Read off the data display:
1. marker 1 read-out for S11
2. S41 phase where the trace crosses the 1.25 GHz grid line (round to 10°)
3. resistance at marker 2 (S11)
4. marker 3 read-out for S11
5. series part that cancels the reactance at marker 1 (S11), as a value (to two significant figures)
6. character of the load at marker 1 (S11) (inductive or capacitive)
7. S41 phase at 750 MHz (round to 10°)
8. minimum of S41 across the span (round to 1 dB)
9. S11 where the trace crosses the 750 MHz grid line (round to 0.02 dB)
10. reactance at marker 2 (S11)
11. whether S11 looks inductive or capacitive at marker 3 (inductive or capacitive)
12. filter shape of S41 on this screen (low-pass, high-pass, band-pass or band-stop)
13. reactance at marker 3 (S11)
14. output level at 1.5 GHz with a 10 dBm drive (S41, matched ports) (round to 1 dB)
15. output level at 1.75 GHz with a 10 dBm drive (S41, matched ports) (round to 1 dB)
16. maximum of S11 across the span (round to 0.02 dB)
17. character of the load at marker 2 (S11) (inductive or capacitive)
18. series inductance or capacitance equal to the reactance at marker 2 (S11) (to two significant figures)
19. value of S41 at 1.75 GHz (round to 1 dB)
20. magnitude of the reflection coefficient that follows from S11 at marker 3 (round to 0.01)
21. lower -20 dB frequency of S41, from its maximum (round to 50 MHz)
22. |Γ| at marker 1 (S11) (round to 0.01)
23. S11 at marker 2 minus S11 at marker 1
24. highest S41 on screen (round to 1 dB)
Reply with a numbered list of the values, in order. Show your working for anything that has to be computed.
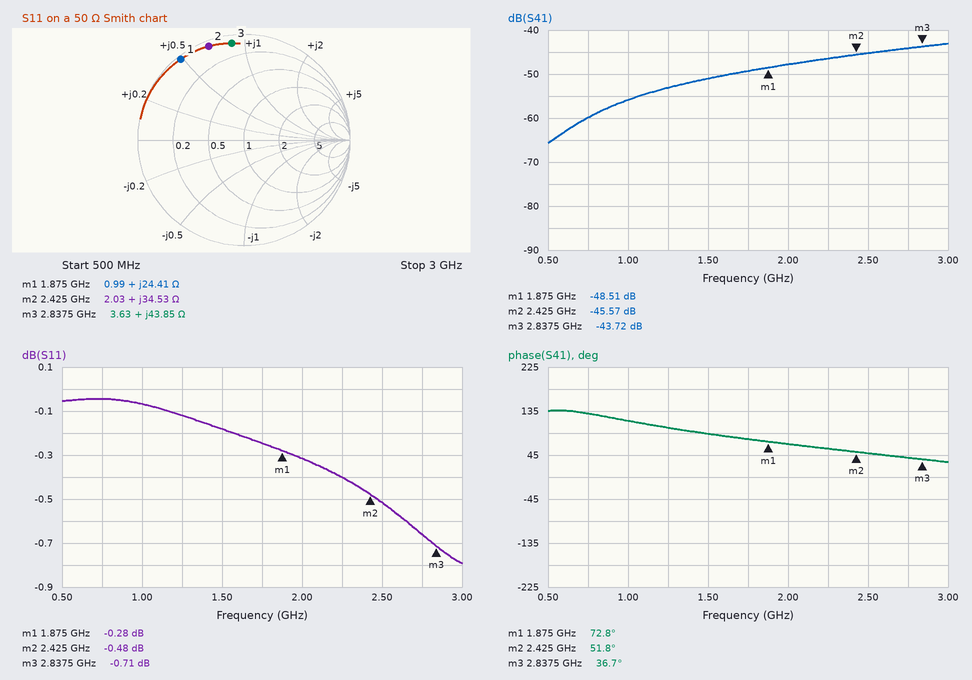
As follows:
1. -0.28 dB
2. 100°
3. 2.03 Ω
4. -0.71 dB
5. C = 1/(2π × 1.875 GHz × 24.41 Ω) ≈ 3.5 pF
6. inductive
7. 130°
8. -66 dB
9. -0.04 dB
10. +34.53 Ω
11. inductive
12. high-pass
13. +43.85 Ω
14. 10 dBm + (-51 dB) = -41 dBm
15. 10 dBm + (-49 dB) = -39 dBm
16. -0.04 dB
17. inductive
18. L = 34.53 Ω/(2π × 2.425 GHz) ≈ 2.3 nH
19. -49 dB
20. 10^(-0.71/20) ≈ 0.92
21. 600 MHz
22. 0.97
23. -0.48 − (-0.28) = -0.20 dB
24. -43 dB
